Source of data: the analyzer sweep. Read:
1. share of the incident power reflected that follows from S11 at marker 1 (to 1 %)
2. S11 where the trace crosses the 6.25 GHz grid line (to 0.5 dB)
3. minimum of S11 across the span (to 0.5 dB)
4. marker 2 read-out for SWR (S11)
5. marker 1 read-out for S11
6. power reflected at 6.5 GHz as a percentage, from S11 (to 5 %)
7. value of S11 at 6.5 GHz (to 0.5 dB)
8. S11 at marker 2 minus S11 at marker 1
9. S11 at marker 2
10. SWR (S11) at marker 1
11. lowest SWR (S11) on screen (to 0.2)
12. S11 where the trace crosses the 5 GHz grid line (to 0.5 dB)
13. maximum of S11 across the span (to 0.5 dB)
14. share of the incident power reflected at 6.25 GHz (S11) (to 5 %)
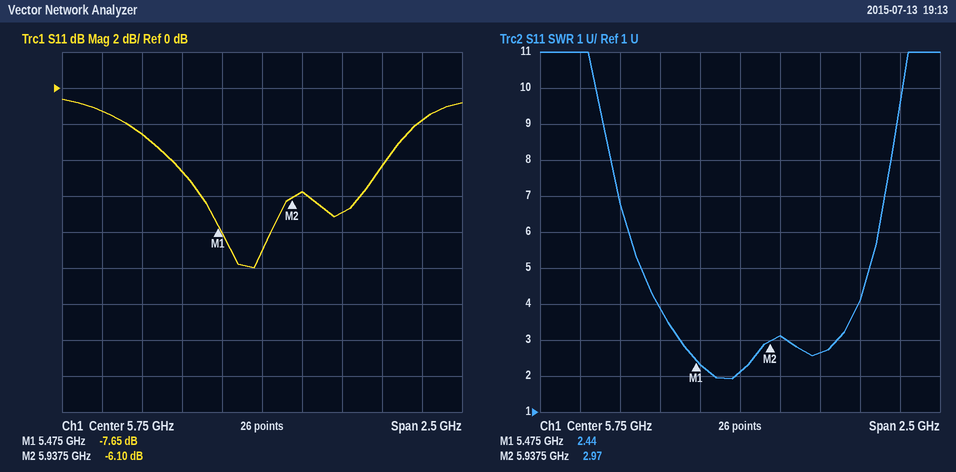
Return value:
17 %
-7.0 dB
-10.0 dB
2.97
-7.65 dB
35 %
-4.5 dB
1.55 dB
-6.10 dB
2.44
2.0
-2.5 dB
-0.5 dB
20 %
